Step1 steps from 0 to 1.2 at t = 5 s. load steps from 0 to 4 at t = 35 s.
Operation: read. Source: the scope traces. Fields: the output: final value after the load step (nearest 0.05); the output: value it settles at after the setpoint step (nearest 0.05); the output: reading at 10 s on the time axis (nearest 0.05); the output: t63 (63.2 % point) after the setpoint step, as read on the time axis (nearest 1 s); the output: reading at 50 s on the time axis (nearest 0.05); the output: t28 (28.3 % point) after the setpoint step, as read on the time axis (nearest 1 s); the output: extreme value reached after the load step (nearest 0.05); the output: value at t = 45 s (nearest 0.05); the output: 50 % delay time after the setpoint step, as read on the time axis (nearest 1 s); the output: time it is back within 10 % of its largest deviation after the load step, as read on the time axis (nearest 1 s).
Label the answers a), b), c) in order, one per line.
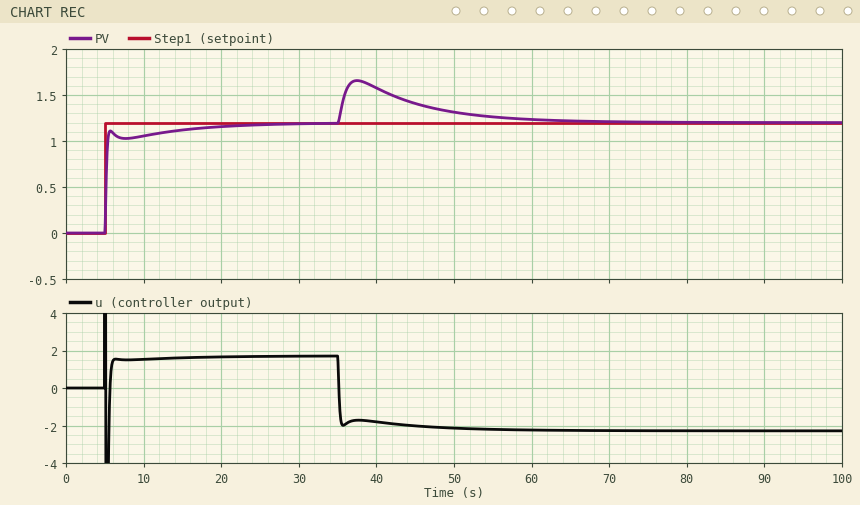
a) 1.20
b) 1.20
c) 1.05
d) 5 s
e) 1.30
f) 5 s
g) 1.65
h) 1.40
i) 5 s
j) 57 s
